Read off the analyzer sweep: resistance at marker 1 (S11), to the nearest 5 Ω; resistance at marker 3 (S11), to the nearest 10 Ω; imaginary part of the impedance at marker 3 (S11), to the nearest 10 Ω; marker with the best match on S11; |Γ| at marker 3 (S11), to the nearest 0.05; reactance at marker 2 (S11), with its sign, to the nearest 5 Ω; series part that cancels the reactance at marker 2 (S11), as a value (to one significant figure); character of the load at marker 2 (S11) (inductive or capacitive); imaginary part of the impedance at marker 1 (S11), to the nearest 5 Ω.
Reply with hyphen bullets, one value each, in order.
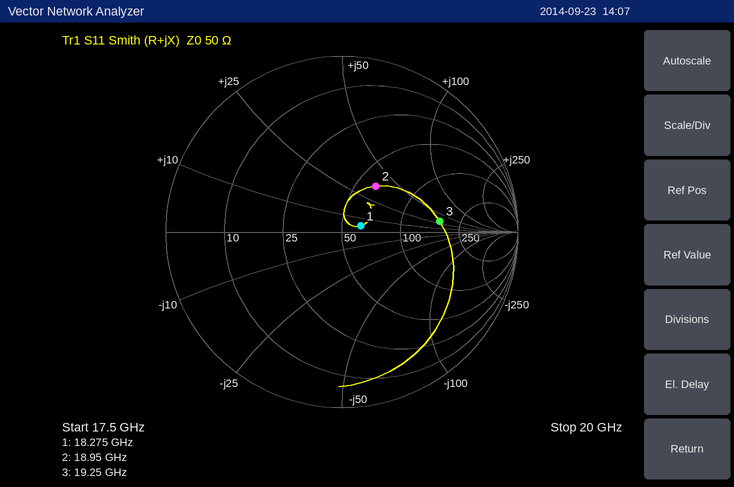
- 60 Ω
- 170 Ω
- +30 Ω
- marker 1
- 0.55
- +35 Ω
- 200 fF
- inductive
- +5 Ω
